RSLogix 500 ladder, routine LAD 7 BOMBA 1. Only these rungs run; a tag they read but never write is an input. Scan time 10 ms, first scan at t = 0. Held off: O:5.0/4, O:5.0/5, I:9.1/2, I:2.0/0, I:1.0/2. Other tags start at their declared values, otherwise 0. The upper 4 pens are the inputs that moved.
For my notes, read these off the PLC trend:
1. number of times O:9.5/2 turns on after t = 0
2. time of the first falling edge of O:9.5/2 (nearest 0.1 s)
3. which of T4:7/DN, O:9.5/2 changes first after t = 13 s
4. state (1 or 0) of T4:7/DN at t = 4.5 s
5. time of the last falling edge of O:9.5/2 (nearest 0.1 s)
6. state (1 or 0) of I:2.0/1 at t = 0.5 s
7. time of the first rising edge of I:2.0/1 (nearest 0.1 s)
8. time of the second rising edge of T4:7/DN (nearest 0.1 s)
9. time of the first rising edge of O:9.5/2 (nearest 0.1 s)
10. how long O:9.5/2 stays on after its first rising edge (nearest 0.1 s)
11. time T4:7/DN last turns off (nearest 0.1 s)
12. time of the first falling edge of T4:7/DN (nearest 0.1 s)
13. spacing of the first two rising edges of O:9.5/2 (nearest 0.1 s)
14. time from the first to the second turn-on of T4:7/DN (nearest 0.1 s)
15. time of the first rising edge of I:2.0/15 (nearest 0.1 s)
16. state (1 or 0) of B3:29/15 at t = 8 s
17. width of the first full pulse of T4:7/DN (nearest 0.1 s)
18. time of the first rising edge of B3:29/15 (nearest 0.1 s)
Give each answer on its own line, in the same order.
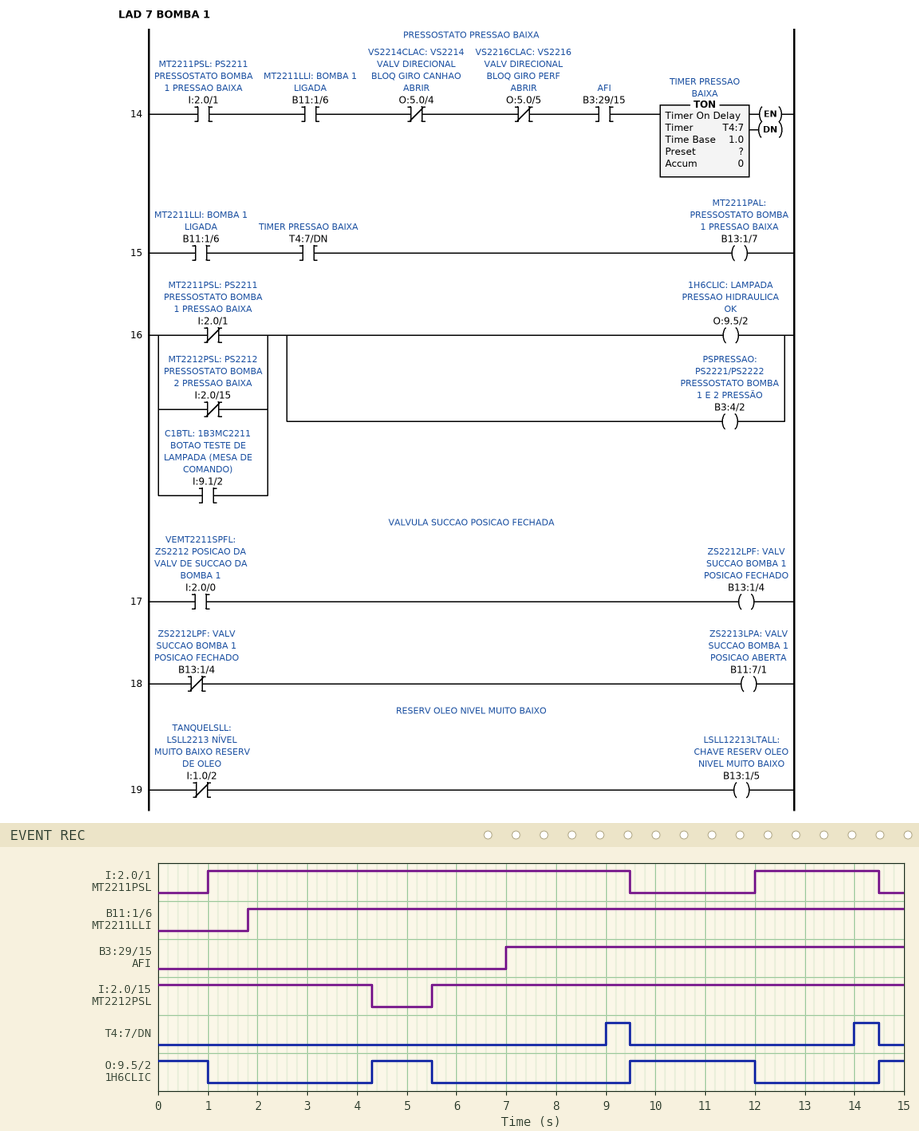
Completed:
3
1.0 s
T4:7/DN
0
12.0 s
0
1.0 s
14.0 s
4.3 s
1.2 s
14.5 s
9.5 s
5.2 s
5.0 s
5.5 s
1
0.5 s
7.0 s
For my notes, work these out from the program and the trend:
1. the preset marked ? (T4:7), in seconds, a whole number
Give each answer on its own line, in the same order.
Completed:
2 s
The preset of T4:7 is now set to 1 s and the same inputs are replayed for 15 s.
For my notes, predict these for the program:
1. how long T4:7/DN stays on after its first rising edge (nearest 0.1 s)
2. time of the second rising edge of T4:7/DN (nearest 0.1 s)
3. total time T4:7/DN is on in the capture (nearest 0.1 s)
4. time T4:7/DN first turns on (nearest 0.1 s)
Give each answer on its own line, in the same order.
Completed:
1.5 s
13.0 s
3.0 s
8.0 s
